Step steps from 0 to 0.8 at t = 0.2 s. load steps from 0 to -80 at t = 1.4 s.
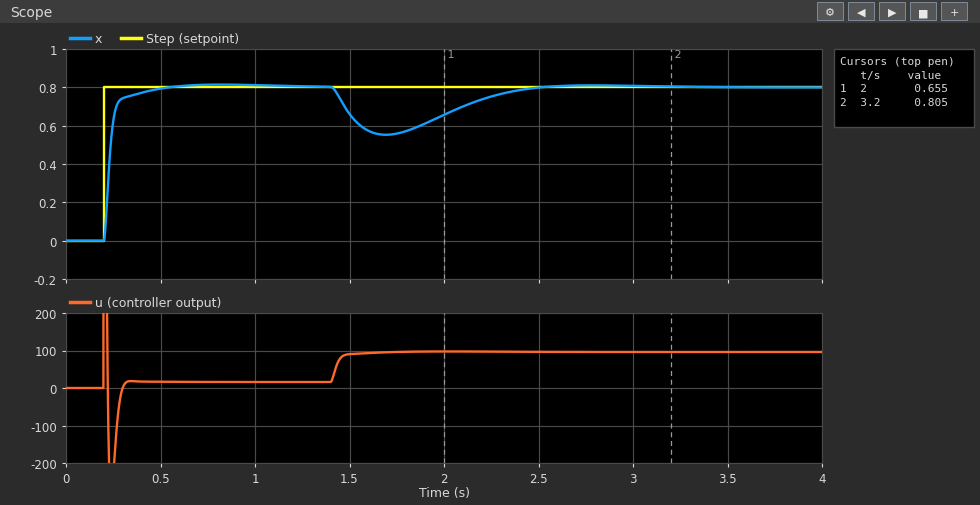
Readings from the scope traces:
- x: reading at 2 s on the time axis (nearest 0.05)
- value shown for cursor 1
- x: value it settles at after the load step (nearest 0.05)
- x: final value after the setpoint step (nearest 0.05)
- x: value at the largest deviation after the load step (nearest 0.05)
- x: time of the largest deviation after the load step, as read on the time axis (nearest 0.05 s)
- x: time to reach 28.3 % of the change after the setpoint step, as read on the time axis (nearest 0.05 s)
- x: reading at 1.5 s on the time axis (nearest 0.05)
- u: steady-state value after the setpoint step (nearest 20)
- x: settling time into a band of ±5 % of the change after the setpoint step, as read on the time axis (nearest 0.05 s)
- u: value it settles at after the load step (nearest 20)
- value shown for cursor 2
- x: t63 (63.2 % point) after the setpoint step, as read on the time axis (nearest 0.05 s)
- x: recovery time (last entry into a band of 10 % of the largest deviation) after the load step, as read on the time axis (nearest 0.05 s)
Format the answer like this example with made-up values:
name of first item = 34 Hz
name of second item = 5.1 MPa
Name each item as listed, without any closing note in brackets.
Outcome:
x: reading at 2 s on the time axis = 0.65
value shown for cursor 1 = 0.655
x: value it settles at after the load step = 0.80
x: final value after the setpoint step = 0.80
x: value at the largest deviation after the load step = 0.55
x: time of the largest deviation after the load step, as read on the time axis = 1.70 s
x: time to reach 28.3 % of the change after the setpoint step, as read on the time axis = 0.20 s
x: reading at 1.5 s on the time axis = 0.65
u: steady-state value after the setpoint step = 20
x: settling time into a band of ±5 % of the change after the setpoint step, as read on the time axis = 0.35 s
u: value it settles at after the load step = 100
value shown for cursor 2 = 0.805
x: t63 (63.2 % point) after the setpoint step, as read on the time axis = 0.25 s
x: recovery time (last entry into a band of 10 % of the largest deviation) after the load step, as read on the time axis = 2.35 s
